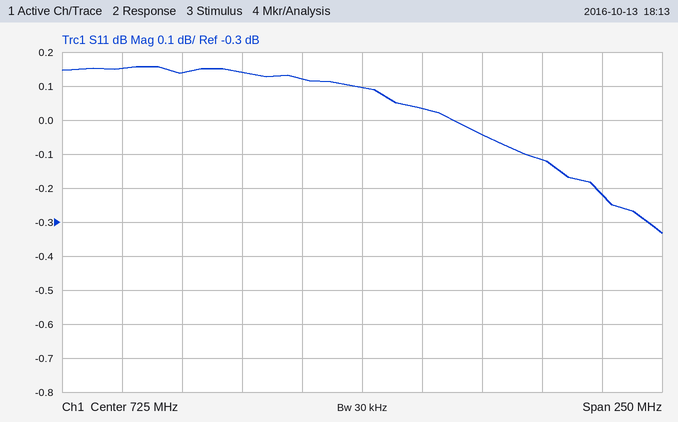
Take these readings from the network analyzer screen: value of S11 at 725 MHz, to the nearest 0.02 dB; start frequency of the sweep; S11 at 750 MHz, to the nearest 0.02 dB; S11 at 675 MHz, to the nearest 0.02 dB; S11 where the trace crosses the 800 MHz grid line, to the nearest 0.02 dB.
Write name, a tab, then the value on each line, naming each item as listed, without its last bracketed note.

value of S11 at 725 MHz, to the nearest 0.02 dB	0.10 dB
start frequency of the sweep	600 MHz
S11 at 750 MHz, to the nearest 0.02 dB	0.04 dB
S11 at 675 MHz, to the nearest 0.02 dB	0.14 dB
S11 where the trace crosses the 800 MHz grid line, to the nearest 0.02 dB	-0.12 dB
